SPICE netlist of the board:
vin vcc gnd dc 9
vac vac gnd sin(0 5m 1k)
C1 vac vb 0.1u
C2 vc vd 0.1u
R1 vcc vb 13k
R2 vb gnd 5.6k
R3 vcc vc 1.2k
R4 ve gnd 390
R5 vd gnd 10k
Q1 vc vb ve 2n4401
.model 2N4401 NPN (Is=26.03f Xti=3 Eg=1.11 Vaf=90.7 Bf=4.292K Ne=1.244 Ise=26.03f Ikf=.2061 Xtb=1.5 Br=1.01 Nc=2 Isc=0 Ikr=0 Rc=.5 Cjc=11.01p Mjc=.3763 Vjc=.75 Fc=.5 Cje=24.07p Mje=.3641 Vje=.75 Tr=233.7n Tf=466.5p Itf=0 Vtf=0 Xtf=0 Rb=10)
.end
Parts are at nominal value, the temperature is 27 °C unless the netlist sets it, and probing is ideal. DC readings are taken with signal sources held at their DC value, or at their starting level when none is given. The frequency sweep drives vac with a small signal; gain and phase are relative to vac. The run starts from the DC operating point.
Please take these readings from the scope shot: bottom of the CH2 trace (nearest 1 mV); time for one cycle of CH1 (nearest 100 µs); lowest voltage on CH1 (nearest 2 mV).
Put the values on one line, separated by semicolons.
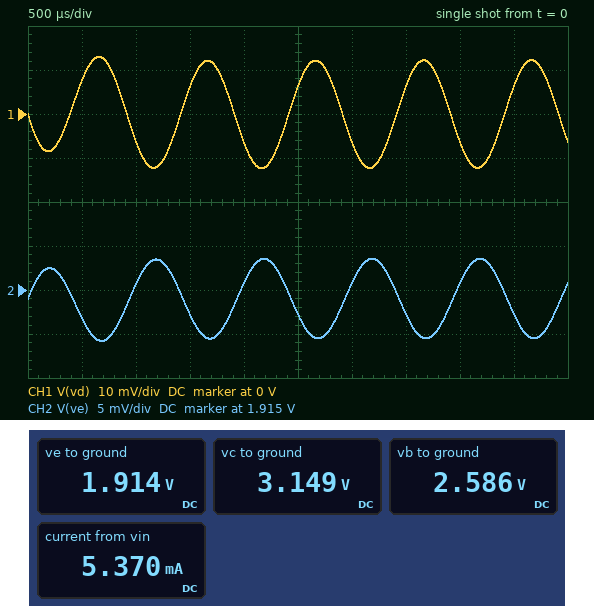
1.909 V; 1.0 ms; -12 mV
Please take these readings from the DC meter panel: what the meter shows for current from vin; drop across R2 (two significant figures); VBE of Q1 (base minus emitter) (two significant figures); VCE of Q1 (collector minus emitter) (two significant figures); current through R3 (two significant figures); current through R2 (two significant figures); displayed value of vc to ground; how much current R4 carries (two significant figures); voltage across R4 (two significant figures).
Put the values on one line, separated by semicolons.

5.370 mA; 2.6 V; 670 mV; 1.2 V; 4.9 mA; 460 µA; 3.149 V; 4.9 mA; 1.9 V
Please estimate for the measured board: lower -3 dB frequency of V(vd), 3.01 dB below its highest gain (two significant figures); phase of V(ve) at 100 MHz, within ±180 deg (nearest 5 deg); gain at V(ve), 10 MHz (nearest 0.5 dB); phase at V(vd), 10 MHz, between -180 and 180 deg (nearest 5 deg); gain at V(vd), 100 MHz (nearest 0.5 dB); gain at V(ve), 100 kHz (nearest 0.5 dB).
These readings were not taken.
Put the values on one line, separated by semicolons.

470 Hz; 0 deg; 0 dB; 135 deg; 1.5 dB; 0 dB
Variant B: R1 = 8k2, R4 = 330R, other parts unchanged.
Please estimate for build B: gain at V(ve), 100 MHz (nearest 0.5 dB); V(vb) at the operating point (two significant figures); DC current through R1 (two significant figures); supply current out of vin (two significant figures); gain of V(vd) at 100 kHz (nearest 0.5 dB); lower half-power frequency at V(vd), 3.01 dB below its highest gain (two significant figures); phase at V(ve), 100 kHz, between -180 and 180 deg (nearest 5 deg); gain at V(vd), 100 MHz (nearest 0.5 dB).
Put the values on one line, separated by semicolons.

-0.5 dB; 2.7 V; 770 µA; 6.5 mA; -4.0 dB; 310 kHz; 5 deg; -0.5 dB
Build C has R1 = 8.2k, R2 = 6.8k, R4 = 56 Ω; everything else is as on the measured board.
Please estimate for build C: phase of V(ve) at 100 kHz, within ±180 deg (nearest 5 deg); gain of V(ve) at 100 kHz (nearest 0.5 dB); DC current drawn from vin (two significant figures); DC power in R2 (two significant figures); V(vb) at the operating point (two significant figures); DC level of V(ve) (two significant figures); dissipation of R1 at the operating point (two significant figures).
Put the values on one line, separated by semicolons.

15 deg; -2.5 dB; 8.0 mA; 190 µW; 1.1 V; 440 mV; 7.5 mW
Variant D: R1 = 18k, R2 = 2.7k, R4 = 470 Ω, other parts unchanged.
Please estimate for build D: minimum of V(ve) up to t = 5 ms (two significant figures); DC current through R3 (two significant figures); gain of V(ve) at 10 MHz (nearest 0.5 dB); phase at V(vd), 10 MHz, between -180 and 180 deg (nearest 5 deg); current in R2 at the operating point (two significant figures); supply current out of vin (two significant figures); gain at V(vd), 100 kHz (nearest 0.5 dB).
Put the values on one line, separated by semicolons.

520 mV; 1.1 mA; -0.5 dB; 150 deg; 430 µA; 1.5 mA; 6.5 dB
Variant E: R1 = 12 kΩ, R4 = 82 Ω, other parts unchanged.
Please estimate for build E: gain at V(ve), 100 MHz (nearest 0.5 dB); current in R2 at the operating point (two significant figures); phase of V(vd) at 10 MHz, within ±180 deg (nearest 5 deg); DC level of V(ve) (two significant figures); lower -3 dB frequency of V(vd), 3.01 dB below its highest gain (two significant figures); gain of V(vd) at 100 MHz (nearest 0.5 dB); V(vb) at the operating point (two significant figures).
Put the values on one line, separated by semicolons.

-1.5 dB; 230 µA; 5 deg; 600 mV; 710 kHz; -1.0 dB; 1.3 V
